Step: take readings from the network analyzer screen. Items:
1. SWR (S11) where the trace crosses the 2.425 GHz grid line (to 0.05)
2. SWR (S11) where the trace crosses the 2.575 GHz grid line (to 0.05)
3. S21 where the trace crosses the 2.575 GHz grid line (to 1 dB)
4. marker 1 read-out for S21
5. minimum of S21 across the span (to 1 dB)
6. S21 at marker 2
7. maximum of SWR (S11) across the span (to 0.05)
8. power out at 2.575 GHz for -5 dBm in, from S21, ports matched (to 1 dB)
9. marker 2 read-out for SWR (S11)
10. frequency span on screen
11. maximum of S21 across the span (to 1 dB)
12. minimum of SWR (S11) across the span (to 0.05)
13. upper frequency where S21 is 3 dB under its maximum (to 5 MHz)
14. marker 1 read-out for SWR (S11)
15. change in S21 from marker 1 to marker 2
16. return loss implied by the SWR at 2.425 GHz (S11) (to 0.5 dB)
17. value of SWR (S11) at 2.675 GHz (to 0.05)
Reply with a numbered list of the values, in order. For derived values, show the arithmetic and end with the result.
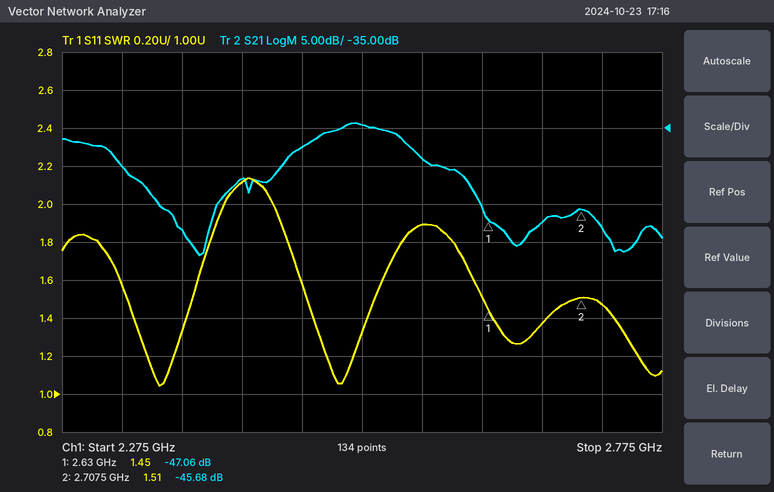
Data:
1. 2.10
2. 1.90
3. -39 dB
4. -47.06 dB
5. -52 dB
6. -45.68 dB
7. 2.15
8. -5 dBm + (-39 dB) = -44 dBm
9. 1.51
10. 500 MHz
11. -34 dB
12. 1.05
13. 2.565 GHz
14. 1.45
15. -45.68 − (-47.06) = 1.38 dB
16. −20 log10((2.1 − 1)/(2.1 + 1)) ≈ 9.0 dB
17. 1.35
